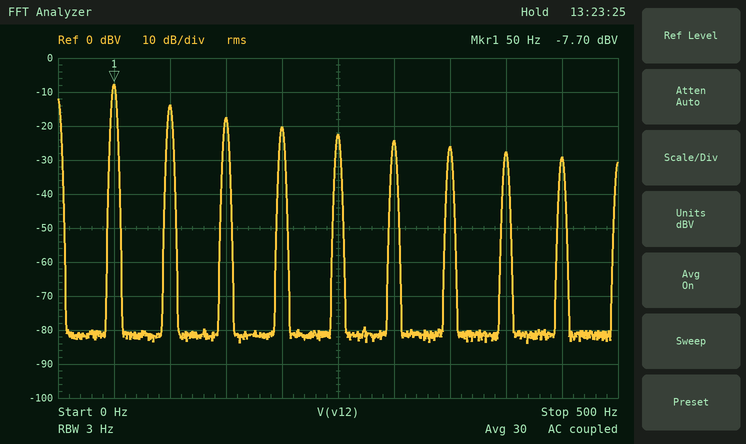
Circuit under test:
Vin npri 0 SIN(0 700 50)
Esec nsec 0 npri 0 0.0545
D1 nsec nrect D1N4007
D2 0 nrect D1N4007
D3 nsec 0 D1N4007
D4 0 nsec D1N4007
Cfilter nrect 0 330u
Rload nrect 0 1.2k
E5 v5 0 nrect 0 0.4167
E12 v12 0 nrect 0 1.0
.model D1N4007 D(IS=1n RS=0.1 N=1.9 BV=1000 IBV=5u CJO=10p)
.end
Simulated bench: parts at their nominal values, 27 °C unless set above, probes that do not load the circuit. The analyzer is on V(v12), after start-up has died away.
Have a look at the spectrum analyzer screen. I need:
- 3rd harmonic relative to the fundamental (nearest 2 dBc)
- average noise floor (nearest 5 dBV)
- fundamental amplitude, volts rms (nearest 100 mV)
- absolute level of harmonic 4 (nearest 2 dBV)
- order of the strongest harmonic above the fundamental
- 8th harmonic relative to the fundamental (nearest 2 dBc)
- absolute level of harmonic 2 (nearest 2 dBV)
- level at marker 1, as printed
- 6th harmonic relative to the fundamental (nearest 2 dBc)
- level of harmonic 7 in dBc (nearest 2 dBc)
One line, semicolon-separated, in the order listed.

-10 dBc; -80 dBV; 400 mV; -20 dBV; 2; -20 dBc; -14 dBV; -7.70 dBV; -16 dBc; -18 dBc
